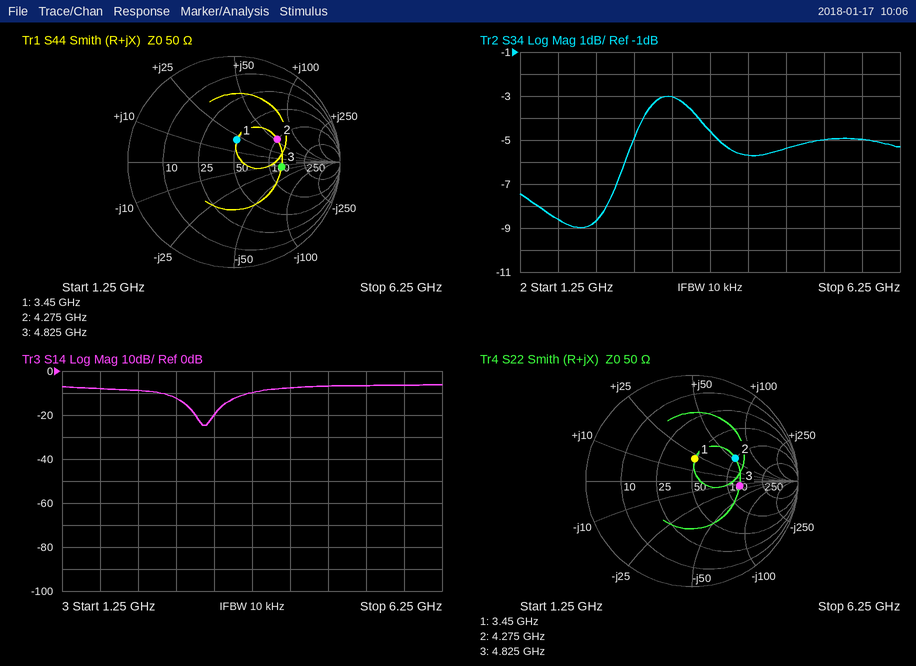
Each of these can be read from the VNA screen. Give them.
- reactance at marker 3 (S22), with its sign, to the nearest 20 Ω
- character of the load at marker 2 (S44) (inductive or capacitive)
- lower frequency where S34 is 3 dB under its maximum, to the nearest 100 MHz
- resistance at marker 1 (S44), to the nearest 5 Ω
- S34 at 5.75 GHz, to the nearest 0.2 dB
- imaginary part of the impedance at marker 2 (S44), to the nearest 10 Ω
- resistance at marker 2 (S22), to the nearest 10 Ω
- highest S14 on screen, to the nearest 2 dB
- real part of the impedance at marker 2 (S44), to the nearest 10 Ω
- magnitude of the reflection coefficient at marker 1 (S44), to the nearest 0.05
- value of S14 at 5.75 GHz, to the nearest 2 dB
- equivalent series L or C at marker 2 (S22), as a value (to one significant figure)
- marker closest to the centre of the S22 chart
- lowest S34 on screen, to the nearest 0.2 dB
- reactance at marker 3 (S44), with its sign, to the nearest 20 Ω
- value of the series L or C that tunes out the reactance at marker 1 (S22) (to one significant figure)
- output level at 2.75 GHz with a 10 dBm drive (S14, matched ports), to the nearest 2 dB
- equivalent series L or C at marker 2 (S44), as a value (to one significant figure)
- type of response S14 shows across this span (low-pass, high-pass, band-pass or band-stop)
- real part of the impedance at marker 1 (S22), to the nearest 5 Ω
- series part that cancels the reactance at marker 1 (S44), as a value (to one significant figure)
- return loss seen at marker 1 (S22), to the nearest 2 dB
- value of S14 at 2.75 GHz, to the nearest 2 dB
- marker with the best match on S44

-20 Ω
inductive
2.6 GHz
50 Ω
-5.0 dB
+50 Ω
100 Ω
-6 dB
100 Ω
0.20
-6 dB
2 nH
marker 1
-9.0 dB
-20 Ω
2 pF
-2 dBm
2 nH
band-stop
50 Ω
2 pF
14 dB
-12 dB
marker 1
